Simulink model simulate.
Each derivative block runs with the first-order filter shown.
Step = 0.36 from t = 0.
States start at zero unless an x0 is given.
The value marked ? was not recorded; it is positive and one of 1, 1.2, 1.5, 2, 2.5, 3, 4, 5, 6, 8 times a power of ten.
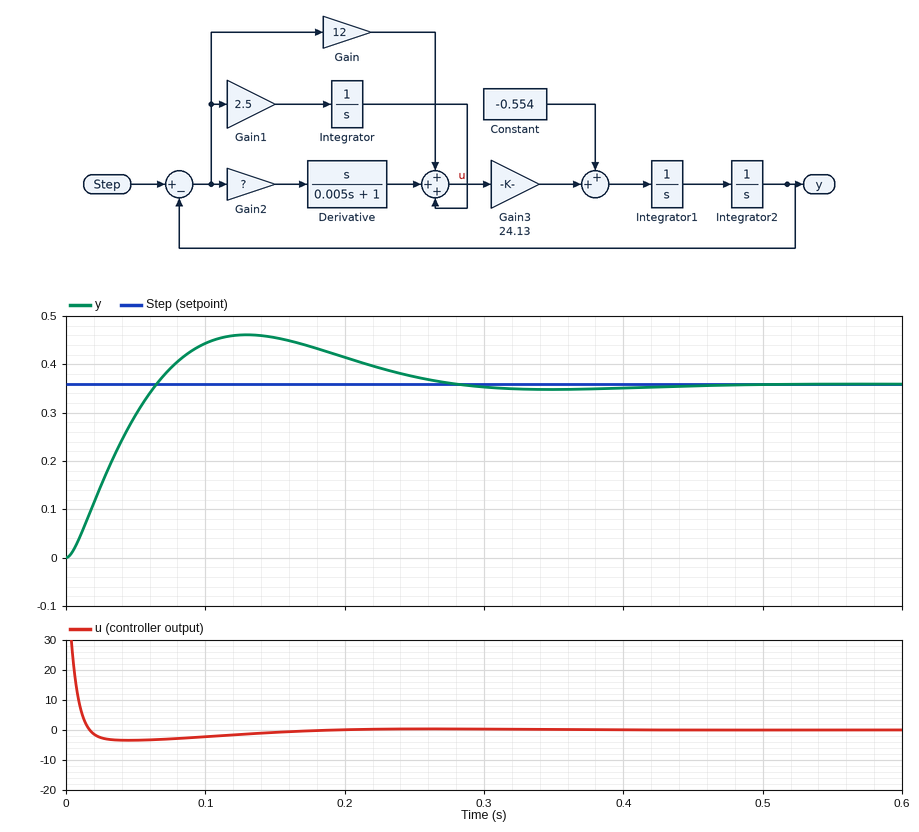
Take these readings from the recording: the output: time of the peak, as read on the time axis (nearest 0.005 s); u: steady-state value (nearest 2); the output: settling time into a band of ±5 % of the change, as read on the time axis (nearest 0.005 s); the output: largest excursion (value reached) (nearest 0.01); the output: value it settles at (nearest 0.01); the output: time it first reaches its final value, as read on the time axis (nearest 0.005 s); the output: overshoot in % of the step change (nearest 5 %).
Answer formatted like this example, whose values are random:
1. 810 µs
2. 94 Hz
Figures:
1. 0.130 s
2. 0
3. 0.245 s
4. 0.46
5. 0.36
6. 0.065 s
7. 30 %
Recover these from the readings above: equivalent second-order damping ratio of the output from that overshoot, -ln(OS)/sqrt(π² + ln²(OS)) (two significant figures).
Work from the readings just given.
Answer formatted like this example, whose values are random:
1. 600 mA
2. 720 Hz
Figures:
1. 0.36
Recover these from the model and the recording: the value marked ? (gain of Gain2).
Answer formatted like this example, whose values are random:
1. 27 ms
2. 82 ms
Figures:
1. 0.8
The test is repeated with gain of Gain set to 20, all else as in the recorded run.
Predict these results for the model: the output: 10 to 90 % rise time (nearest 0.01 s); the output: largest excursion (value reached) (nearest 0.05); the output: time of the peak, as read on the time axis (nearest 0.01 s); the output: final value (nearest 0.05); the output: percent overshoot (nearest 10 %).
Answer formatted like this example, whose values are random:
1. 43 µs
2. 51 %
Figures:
1. 0.04 s
2. 0.50
3. 0.11 s
4. 0.35
5. 40 %
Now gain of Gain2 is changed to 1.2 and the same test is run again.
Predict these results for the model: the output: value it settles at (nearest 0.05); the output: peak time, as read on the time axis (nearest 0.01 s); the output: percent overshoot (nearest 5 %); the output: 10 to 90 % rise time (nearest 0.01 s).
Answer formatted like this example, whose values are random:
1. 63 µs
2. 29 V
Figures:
1. 0.35
2. 0.11 s
3. 20 %
4. 0.04 s
